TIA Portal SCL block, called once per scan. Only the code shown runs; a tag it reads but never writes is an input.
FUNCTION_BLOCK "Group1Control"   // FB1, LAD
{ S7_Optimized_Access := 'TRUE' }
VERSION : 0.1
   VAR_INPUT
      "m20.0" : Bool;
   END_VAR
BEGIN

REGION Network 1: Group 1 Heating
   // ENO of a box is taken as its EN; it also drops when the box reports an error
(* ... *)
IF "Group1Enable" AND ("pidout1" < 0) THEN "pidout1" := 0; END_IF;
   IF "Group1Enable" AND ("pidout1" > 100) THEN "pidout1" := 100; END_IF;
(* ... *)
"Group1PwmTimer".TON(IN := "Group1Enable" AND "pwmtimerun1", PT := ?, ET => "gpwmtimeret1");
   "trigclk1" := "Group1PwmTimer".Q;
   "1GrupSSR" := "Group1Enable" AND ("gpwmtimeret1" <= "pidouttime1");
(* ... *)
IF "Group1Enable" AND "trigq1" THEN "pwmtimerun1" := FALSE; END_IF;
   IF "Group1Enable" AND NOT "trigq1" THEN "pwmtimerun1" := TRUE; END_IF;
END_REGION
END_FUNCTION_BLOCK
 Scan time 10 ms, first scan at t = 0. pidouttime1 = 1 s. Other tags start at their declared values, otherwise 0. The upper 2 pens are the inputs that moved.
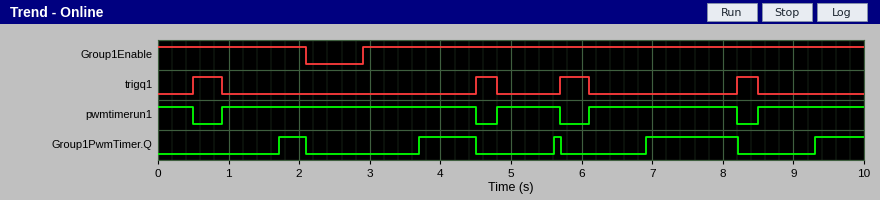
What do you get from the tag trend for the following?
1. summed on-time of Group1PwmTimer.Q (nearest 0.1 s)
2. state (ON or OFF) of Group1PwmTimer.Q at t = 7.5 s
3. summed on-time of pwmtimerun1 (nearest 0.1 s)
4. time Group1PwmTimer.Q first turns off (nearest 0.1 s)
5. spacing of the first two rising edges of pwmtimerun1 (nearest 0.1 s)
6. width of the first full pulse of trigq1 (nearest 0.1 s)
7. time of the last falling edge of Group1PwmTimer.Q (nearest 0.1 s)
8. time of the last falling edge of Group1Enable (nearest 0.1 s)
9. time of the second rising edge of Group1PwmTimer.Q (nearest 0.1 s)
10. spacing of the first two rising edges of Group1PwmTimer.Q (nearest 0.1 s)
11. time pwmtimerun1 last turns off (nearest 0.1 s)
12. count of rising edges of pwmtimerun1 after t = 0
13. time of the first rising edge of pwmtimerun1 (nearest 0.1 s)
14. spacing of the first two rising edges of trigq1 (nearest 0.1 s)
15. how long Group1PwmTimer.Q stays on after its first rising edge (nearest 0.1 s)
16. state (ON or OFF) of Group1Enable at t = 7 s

3.3 s
ON
8.6 s
2.1 s
3.9 s
0.4 s
8.2 s
2.1 s
3.7 s
2.0 s
8.2 s
4
0.9 s
4.0 s
0.4 s
ON
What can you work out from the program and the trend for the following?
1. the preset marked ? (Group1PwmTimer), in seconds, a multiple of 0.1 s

0.8 s
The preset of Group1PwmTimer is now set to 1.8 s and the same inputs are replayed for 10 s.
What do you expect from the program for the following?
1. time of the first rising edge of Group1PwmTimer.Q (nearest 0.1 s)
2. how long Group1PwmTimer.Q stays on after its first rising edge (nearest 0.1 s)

7.9 s
0.3 s
